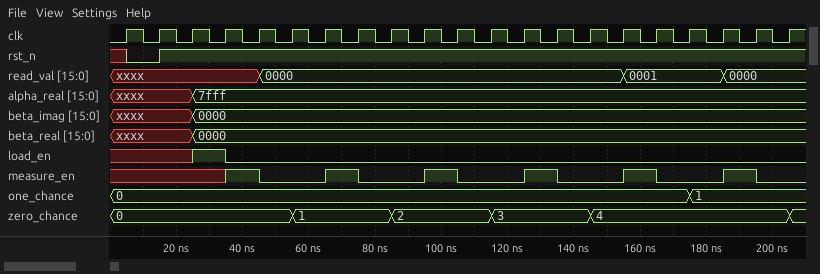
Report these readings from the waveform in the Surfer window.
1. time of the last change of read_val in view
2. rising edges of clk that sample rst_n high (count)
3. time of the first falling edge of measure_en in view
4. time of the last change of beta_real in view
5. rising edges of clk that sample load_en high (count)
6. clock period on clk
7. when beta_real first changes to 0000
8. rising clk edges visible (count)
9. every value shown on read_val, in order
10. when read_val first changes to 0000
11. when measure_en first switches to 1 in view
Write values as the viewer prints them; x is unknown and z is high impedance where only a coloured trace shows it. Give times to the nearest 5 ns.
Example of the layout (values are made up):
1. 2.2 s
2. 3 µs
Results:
1. 185 ns
2. 19
3. 45 ns
4. 25 ns
5. 1
6. 10 ns
7. 25 ns
8. 21
9. xxxx, 0000, 0001, 0000
10. 45 ns
11. 35 ns
